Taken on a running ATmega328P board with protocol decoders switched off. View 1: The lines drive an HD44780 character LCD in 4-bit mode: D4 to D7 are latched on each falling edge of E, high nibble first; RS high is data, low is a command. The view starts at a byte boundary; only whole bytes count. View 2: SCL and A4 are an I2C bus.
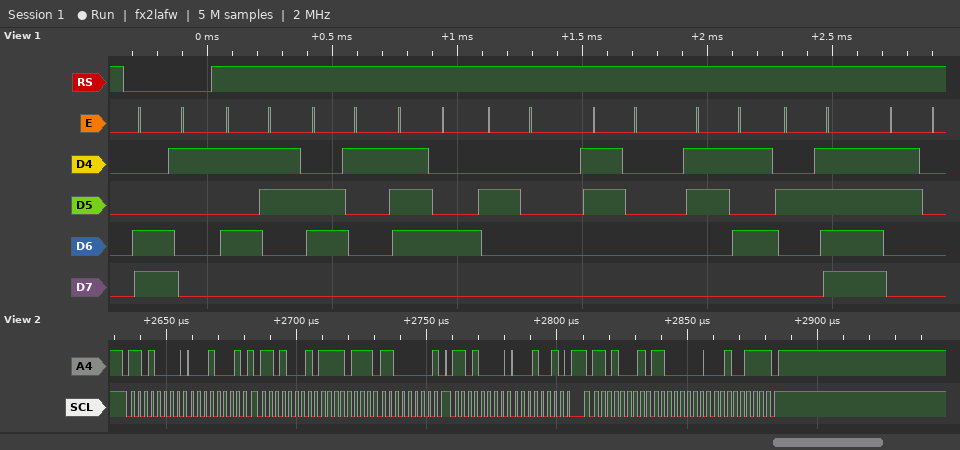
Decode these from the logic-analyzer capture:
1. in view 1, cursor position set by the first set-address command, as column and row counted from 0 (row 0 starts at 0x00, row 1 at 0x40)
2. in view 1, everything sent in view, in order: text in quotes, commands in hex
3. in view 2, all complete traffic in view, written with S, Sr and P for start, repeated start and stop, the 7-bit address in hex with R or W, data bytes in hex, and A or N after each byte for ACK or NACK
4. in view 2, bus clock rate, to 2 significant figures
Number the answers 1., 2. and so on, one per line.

1. column 1, row 1
2. 0xC1 "Sat 05/0"
3. S 68W A 11 A Sr 68R A F7 A C0 N P S 68W A 12 A Sr 68R A C0 A 27 N P
4. 400 kHz
